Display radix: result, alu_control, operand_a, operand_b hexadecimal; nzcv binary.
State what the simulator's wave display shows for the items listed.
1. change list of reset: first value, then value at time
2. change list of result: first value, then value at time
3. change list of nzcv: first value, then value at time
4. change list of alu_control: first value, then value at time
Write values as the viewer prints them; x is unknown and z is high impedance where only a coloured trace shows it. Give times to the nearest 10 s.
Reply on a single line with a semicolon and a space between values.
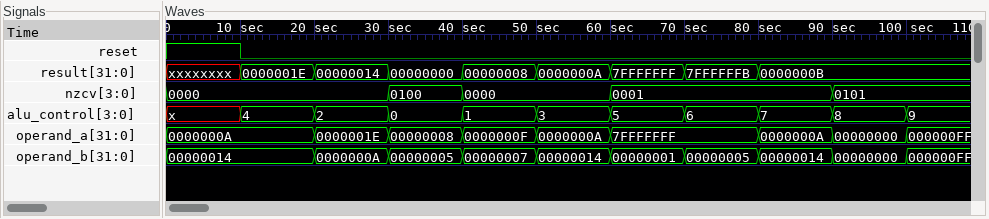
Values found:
1, 0 at 10 s; xxxxxxxx, 0000001E at 10 s, 00000014 at 20 s, 00000000 at 30 s, 00000008 at 40 s, 0000000A at 50 s, 7FFFFFFF at 60 s, 7FFFFFFB at 70 s, 0000000B at 80 s; 0000, 0100 at 30 s, 0000 at 40 s, 0001 at 60 s, 0101 at 90 s; x, 4 at 10 s, 2 at 20 s, 0 at 30 s, 1 at 40 s, 3 at 50 s, 5 at 60 s, 6 at 70 s, 7 at 80 s, 8 at 90 s, 9 at 100 s
